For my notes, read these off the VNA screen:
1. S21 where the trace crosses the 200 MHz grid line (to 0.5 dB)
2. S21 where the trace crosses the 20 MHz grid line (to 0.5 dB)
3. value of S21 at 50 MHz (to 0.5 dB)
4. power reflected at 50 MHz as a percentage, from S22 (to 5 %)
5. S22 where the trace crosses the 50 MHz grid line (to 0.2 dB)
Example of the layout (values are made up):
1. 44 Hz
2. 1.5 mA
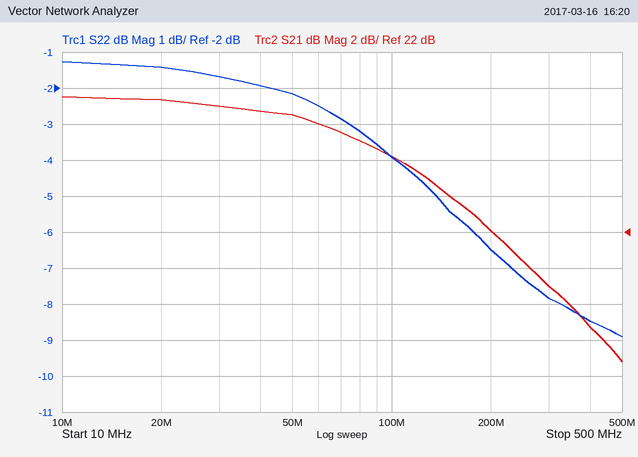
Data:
1. 22.0 dB
2. 29.5 dB
3. 28.5 dB
4. 60 %
5. -2.2 dB
